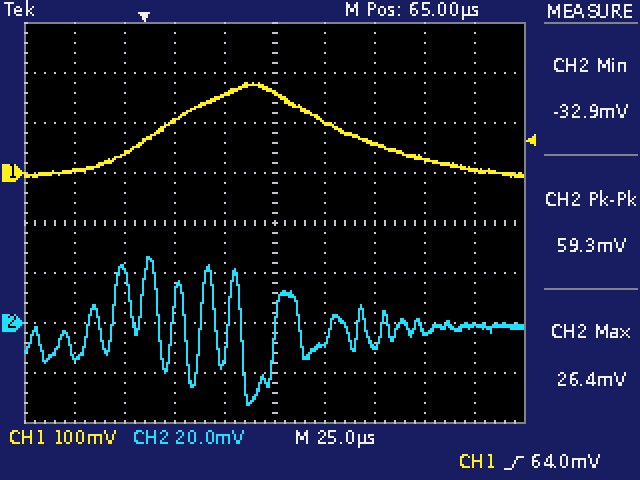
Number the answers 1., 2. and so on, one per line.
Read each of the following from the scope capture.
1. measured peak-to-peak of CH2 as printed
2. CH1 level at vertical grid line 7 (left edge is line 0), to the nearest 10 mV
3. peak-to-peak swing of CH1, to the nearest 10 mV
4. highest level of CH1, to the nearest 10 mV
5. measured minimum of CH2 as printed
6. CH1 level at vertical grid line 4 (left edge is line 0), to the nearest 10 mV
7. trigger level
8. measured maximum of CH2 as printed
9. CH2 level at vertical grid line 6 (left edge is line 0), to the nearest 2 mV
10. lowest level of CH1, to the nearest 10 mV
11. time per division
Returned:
1. 59.3 mV
2. 60 mV
3. 190 mV
4. 180 mV
5. -32.9 mV
6. 160 mV
7. 64.0 mV
8. 26.4 mV
9. -8 mV
10. -10 mV
11. 25 µs
